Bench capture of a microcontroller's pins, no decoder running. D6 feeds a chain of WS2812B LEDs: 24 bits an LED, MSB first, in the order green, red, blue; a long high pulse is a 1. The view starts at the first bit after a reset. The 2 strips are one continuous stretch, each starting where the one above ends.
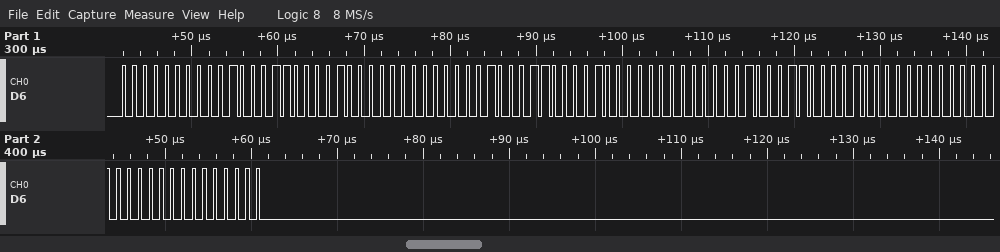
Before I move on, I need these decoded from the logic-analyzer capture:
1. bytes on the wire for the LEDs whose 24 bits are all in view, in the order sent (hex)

00 23 08 00 23 08 00 23 08 00 00 00
